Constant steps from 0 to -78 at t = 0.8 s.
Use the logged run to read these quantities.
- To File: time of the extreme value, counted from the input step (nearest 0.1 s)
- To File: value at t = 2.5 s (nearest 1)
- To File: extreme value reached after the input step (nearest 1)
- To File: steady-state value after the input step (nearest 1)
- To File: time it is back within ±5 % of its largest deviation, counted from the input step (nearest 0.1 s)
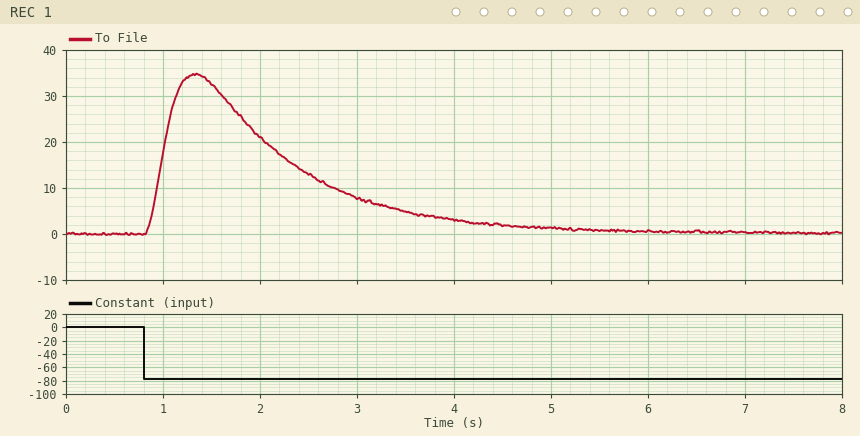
0.5 s
13
35
0
3.7 s
